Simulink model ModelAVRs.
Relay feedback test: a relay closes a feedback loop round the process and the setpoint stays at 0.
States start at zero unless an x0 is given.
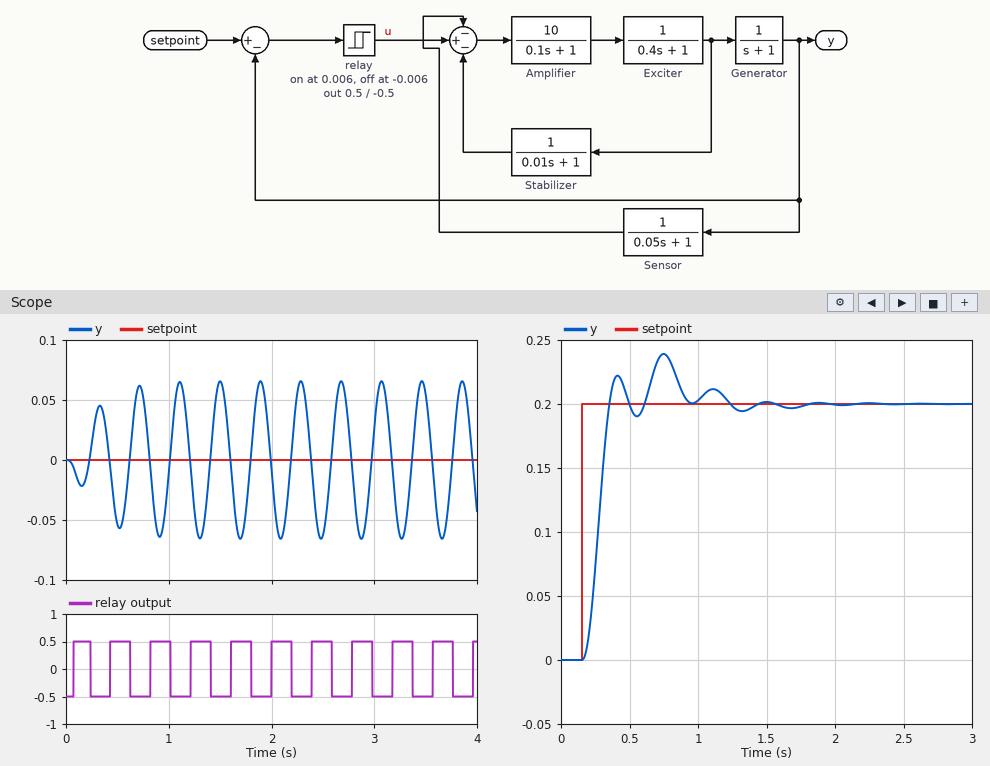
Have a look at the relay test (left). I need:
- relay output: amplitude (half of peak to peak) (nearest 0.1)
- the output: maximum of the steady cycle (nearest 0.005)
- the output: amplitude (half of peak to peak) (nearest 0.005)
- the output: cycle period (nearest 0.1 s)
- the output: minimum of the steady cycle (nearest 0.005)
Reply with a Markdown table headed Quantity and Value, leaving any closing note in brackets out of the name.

| Quantity | Value |
|---|---|
| relay output: amplitude (half of peak to peak) | 0.5 |
| the output: maximum of the steady cycle | 0.065 |
| the output: amplitude (half of peak to peak) | 0.065 |
| the output: cycle period | 0.4 s |
| the output: minimum of the steady cycle | -0.065 |
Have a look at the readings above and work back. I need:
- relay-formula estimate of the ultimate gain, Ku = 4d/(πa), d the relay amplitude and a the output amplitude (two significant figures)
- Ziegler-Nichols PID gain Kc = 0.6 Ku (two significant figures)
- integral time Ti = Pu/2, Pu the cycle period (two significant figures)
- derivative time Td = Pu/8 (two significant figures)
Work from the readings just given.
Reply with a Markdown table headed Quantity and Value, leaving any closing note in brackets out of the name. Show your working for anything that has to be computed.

| Quantity | Value |
|---|---|
| relay-formula estimate of the ultimate gain, Ku = 4d/(πa), d the relay amplitude and a the output amplitude | 4 × 0.5 / (π × 0.065) = 9.8 |
| Ziegler-Nichols PID gain Kc = 0.6 Ku | 0.6 × 9.8 = 5.9 |
| integral time Ti = Pu/2, Pu the cycle period | 0.4 / 2 = 0.20 s |
| derivative time Td = Pu/8 | 0.4 / 8 = 0.050 s |
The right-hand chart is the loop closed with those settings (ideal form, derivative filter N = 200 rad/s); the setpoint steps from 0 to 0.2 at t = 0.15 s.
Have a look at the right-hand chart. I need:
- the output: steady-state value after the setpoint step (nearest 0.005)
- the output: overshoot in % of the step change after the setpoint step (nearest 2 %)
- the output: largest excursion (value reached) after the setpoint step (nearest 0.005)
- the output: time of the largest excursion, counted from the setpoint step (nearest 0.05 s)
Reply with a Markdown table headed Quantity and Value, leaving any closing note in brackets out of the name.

| Quantity | Value |
|---|---|
| the output: steady-state value after the setpoint step | 0.200 |
| the output: overshoot in % of the step change after the setpoint step | 20 % |
| the output: largest excursion (value reached) after the setpoint step | 0.240 |
| the output: time of the largest excursion, counted from the setpoint step | 0.60 s |
